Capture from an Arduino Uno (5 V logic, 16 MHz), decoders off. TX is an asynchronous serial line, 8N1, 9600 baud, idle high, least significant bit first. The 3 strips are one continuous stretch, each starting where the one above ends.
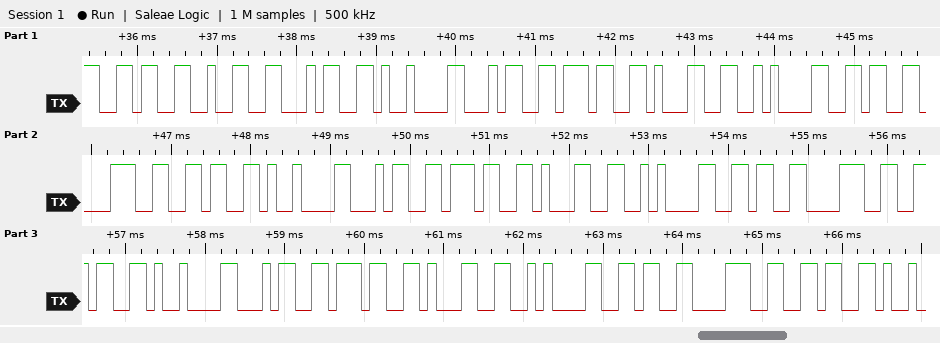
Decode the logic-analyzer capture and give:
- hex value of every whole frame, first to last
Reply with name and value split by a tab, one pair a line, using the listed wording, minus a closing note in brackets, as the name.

hex value of every whole frame, first to last	36 32 34 09 34 37 31 0A 36 38 36 09 34 37 31 0A 36 38 36 09 34 37 31 0A 36 38 36
